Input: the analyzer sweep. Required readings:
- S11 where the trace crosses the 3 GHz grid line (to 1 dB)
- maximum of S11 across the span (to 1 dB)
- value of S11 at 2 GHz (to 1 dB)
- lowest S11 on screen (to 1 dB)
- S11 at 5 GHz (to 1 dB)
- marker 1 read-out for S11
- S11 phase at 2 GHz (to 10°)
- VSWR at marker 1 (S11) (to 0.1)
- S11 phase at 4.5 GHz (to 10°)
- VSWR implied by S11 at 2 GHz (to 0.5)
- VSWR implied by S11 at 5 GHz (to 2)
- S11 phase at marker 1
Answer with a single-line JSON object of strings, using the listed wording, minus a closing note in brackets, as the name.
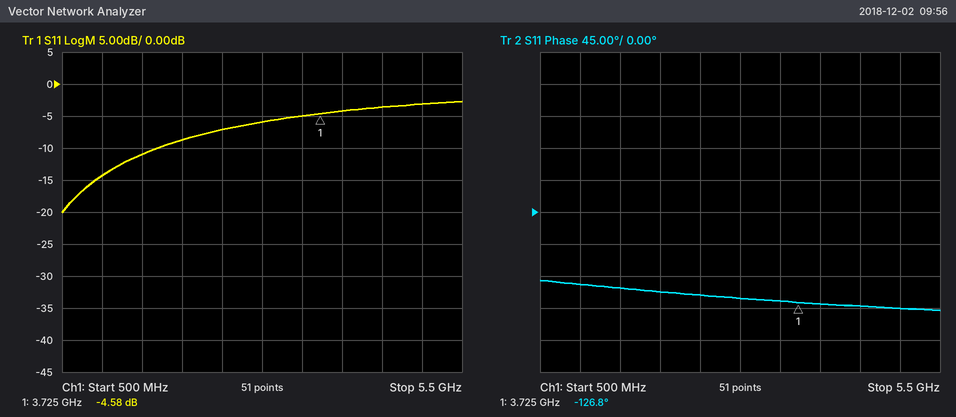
{"S11 where the trace crosses the 3 GHz grid line": "-6 dB", "maximum of S11 across the span": "-3 dB", "value of S11 at 2 GHz": "-9 dB", "lowest S11 on screen": "-20 dB", "S11 at 5 GHz": "-3 dB", "marker 1 read-out for S11": "-4.58 dB", "S11 phase at 2 GHz": "-110°", "VSWR at marker 1 (S11)": "3.9", "S11 phase at 4.5 GHz": "-130°", "VSWR implied by S11 at 2 GHz": "2.0", "VSWR implied by S11 at 5 GHz": "6", "S11 phase at marker 1": "-126.8°"}
